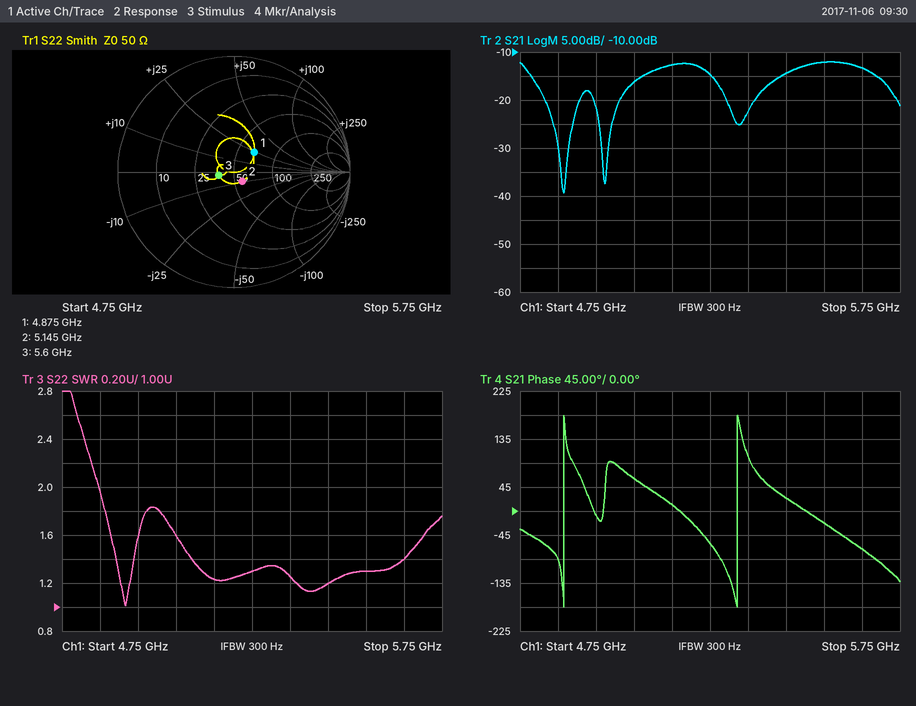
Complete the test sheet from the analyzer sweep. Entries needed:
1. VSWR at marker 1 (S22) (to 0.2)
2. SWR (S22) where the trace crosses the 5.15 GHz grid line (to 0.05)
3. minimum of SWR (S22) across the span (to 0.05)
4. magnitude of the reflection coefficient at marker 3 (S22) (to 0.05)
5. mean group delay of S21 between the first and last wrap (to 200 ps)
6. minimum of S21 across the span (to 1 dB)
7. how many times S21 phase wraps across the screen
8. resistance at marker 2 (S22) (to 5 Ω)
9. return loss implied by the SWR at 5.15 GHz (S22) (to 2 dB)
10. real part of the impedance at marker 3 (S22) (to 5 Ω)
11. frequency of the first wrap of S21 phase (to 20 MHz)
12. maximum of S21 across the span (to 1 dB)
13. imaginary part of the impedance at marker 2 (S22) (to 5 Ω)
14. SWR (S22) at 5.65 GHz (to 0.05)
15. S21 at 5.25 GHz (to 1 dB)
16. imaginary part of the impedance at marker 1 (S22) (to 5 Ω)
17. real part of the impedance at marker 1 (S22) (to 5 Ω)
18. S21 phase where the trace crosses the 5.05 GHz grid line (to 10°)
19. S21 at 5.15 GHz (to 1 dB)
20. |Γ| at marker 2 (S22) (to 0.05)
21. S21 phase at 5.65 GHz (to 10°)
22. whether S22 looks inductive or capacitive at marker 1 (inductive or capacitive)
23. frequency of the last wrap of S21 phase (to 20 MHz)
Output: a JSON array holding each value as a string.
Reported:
["1.6", "1.25", "1.00", "0.15", "2.2 ns", "-39 dB", "2", "55 Ω", "20 dB", "40 Ω", "4.86 GHz", "-12 dB", "-10 Ω", "1.40", "-15 dB", "+25 Ω", "65 Ω", "60°", "-13 dB", "0.10", "-70°", "inductive", "5.32 GHz"]
